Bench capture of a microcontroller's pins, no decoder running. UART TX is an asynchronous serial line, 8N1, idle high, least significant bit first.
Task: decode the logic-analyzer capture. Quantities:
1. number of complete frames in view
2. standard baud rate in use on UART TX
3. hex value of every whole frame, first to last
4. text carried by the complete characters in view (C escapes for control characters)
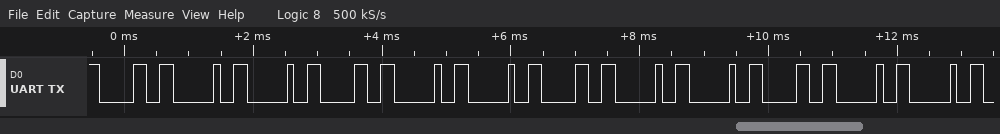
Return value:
12
9600 baud
0x30 0x20 0x20 0x30 0x20 0x20 0x30 0x20 0x20 0x30 0x20 0x20
"0  0  0  0  "
